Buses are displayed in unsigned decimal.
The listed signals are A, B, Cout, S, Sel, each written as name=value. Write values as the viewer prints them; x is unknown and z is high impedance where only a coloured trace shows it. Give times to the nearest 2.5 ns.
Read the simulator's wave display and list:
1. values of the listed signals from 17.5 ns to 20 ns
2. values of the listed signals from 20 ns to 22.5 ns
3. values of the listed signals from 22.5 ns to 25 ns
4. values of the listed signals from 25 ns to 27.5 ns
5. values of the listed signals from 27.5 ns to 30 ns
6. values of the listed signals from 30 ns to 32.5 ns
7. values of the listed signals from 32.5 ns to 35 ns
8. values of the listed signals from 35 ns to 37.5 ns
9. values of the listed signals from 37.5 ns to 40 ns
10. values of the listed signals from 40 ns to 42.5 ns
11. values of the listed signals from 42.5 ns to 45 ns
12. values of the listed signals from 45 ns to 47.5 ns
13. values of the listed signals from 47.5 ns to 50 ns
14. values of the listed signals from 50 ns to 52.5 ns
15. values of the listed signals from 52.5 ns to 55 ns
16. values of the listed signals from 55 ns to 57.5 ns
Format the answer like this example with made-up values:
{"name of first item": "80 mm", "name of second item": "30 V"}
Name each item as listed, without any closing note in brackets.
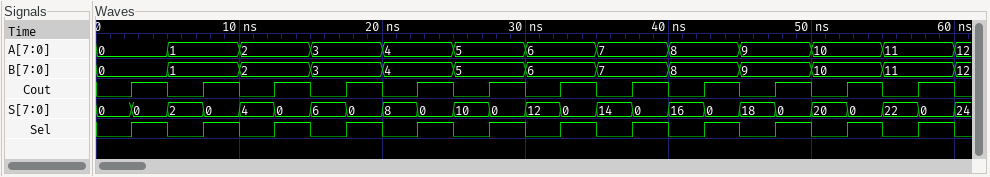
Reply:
{"values of the listed signals from 17.5 ns to 20 ns": "A=3, B=3, Cout=1, S=0, Sel=1", "values of the listed signals from 20 ns to 22.5 ns": "A=4, B=4, Cout=0, S=8, Sel=0", "values of the listed signals from 22.5 ns to 25 ns": "A=4, B=4, Cout=1, S=0, Sel=1", "values of the listed signals from 25 ns to 27.5 ns": "A=5, B=5, Cout=0, S=10, Sel=0", "values of the listed signals from 27.5 ns to 30 ns": "A=5, B=5, Cout=1, S=0, Sel=1", "values of the listed signals from 30 ns to 32.5 ns": "A=6, B=6, Cout=0, S=12, Sel=0", "values of the listed signals from 32.5 ns to 35 ns": "A=6, B=6, Cout=1, S=0, Sel=1", "values of the listed signals from 35 ns to 37.5 ns": "A=7, B=7, Cout=0, S=14, Sel=0", "values of the listed signals from 37.5 ns to 40 ns": "A=7, B=7, Cout=1, S=0, Sel=1", "values of the listed signals from 40 ns to 42.5 ns": "A=8, B=8, Cout=0, S=16, Sel=0", "values of the listed signals from 42.5 ns to 45 ns": "A=8, B=8, Cout=1, S=0, Sel=1", "values of the listed signals from 45 ns to 47.5 ns": "A=9, B=9, Cout=0, S=18, Sel=0", "values of the listed signals from 47.5 ns to 50 ns": "A=9, B=9, Cout=1, S=0, Sel=1", "values of the listed signals from 50 ns to 52.5 ns": "A=10, B=10, Cout=0, S=20, Sel=0", "values of the listed signals from 52.5 ns to 55 ns": "A=10, B=10, Cout=1, S=0, Sel=1", "values of the listed signals from 55 ns to 57.5 ns": "A=11, B=11, Cout=0, S=22, Sel=0"}
